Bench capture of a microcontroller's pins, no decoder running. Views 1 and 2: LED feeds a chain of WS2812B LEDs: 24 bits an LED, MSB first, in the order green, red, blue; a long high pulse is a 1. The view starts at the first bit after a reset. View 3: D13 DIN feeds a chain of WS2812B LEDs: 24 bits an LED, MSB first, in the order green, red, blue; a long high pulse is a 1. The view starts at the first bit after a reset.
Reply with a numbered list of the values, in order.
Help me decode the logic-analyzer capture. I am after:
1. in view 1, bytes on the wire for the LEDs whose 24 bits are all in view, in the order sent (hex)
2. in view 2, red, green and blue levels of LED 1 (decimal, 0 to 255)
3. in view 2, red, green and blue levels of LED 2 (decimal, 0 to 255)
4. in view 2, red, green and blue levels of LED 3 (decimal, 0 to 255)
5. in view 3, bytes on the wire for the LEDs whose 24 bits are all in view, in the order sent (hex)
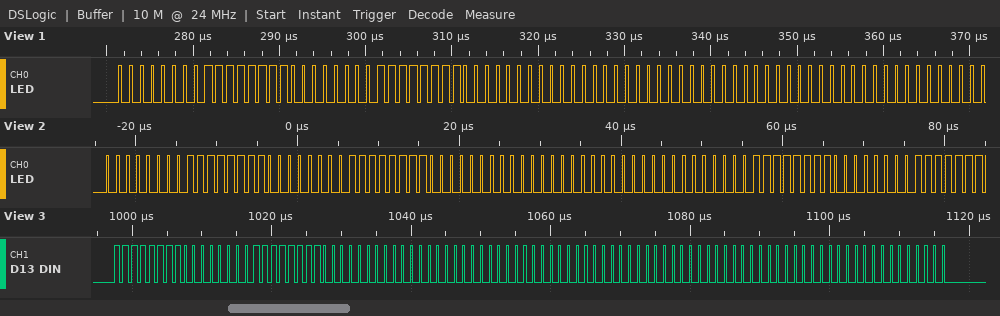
1. 00 FF 00 FF 00 00 00 00 00
2. 255, 0, 0
3. 0, 255, 0
4. 0, 0, 255
5. FF 00 FF 00 00 00 00 00 00 00 00 00
